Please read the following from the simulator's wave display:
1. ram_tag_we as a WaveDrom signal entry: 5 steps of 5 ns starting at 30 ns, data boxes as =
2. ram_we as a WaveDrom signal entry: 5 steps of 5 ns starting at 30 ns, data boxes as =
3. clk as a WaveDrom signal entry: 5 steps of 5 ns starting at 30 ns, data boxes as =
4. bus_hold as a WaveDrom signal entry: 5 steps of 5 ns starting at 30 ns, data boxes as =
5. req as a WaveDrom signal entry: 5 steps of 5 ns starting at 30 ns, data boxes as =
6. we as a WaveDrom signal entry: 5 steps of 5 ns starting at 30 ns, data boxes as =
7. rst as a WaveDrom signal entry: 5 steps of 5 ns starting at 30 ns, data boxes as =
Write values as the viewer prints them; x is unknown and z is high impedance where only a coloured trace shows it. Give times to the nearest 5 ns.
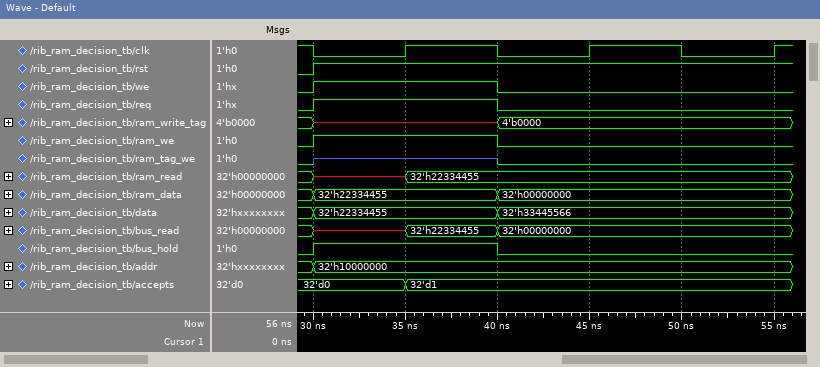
{name: 'ram_tag_we', wave: 'z.0..'}
{name: 'ram_we', wave: '1.0..'}
{name: 'clk', wave: '01010'}
{name: 'bus_hold', wave: '1.0..'}
{name: 'req', wave: '1.0..'}
{name: 'we', wave: '1.0..'}
{name: 'rst', wave: '1....'}
